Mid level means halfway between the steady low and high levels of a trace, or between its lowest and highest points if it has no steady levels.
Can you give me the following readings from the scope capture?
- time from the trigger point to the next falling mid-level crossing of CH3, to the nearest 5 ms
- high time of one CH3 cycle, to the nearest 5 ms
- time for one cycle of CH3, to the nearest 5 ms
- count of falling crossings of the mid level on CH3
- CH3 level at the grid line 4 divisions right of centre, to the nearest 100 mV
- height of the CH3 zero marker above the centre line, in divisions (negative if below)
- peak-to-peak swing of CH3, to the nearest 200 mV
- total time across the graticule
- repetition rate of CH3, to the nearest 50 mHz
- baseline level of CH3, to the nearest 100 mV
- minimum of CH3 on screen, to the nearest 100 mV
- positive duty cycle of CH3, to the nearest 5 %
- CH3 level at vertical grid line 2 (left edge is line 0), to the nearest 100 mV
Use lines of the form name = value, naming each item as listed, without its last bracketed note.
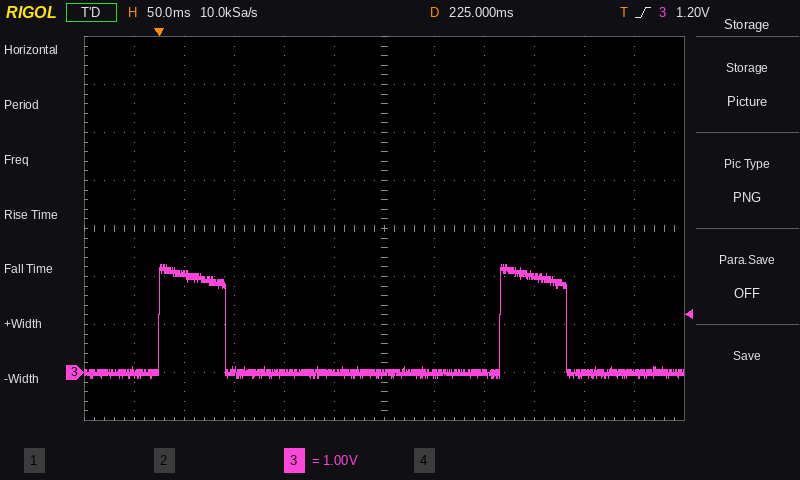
time from the trigger point to the next falling mid-level crossing of CH3, to the nearest 5 ms = 65 ms
high time of one CH3 cycle, to the nearest 5 ms = 65 ms
time for one cycle of CH3, to the nearest 5 ms = 340 ms
count of falling crossings of the mid level on CH3 = 2
CH3 level at the grid line 4 divisions right of centre, to the nearest 100 mV = 0.0 V
height of the CH3 zero marker above the centre line, in divisions = -3.0 div
peak-to-peak swing of CH3, to the nearest 200 mV = 2.4 V
total time across the graticule = 600 ms
repetition rate of CH3, to the nearest 50 mHz = 2.95 Hz
baseline level of CH3, to the nearest 100 mV = 0.0 V
minimum of CH3 on screen, to the nearest 100 mV = -100 mV
positive duty cycle of CH3, to the nearest 5 % = 20 %
CH3 level at vertical grid line 2 (left edge is line 0), to the nearest 100 mV = 2.0 V
